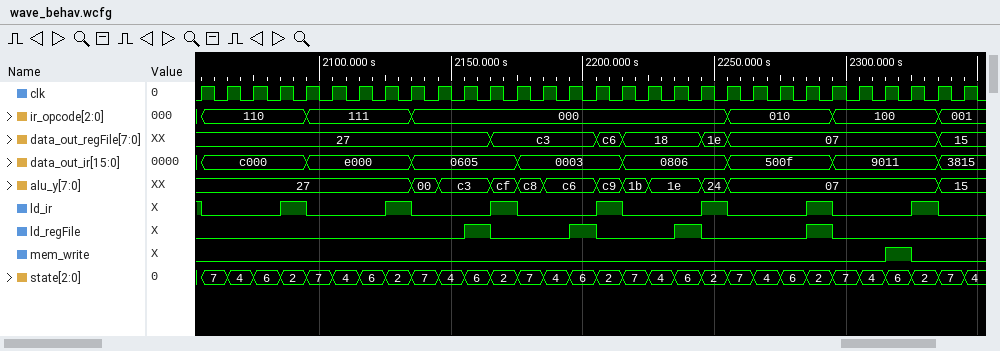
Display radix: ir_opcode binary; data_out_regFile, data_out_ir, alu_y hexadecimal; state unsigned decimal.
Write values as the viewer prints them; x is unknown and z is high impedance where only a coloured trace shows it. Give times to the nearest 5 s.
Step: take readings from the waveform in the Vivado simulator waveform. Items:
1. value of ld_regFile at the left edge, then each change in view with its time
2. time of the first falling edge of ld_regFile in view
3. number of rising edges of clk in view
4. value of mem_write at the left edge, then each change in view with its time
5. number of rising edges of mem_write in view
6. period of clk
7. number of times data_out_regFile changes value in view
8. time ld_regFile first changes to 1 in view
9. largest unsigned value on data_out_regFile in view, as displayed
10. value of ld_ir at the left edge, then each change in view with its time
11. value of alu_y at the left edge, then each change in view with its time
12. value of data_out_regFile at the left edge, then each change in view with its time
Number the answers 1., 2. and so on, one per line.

1. 0, 1 at 2155 s, 0 at 2165 s, 1 at 2195 s, 0 at 2205 s, 1 at 2235 s, 0 at 2245 s, 1 at 2285 s, 0 at 2295 s
2. 2165 s
3. 30
4. 0, 1 at 2315 s, 0 at 2325 s
5. 1
6. 10 s
7. 6
8. 2155 s
9. c6
10. 1, 0 at 2055 s, 1 at 2085 s, 0 at 2095 s, 1 at 2125 s, 0 at 2135 s, 1 at 2165 s, 0 at 2175 s, 1 at 2205 s, 0 at 2215 s, 1 at 2245 s, 0 at 2255 s, 1 at 2285 s, 0 at 2295 s, 1 at 2325 s, 0 at 2335 s
11. 27, 00 at 2135 s, c3 at 2145 s, cf at 2165 s, c8 at 2175 s, c6 at 2185 s, c9 at 2205 s, 1b at 2215 s, 1e at 2225 s, 24 at 2245 s, 07 at 2255 s, 15 at 2335 s
12. 27, c3 at 2165 s, c6 at 2205 s, 18 at 2215 s, 1e at 2245 s, 07 at 2255 s, 15 at 2335 s
